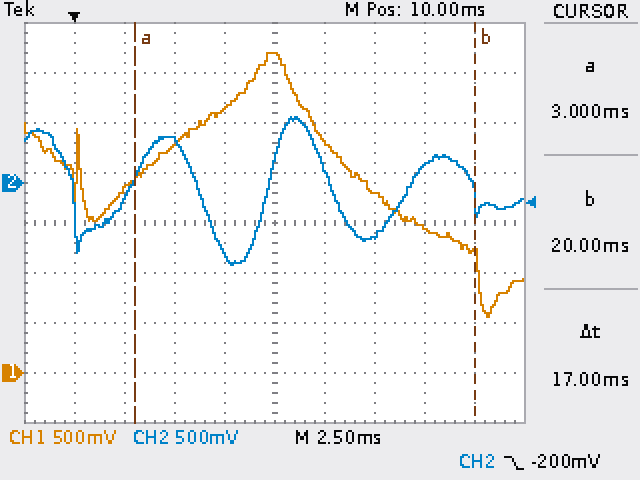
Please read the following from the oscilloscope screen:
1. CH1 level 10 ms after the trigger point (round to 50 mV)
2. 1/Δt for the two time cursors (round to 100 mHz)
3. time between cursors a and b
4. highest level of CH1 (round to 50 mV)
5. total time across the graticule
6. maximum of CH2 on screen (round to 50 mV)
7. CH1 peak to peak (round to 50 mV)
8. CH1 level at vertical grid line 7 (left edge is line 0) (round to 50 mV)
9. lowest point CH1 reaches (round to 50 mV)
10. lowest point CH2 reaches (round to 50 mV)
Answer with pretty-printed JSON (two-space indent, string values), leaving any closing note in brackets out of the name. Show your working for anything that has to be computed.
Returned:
{
  "CH1 level 10 ms after the trigger point": "3.20 V",
  "1/Δt for the two time cursors": "1 / 17 ms ≈ 58.8 Hz",
  "time between cursors a and b": "17 ms",
  "highest level of CH1": "3.20 V",
  "total time across the graticule": "25 ms",
  "maximum of CH2 on screen": "650 mV",
  "CH1 peak to peak": "3.20 V − (550 mV) = 2.65 V",
  "CH1 level at vertical grid line 7 (left edge is line 0)": "1.80 V",
  "lowest point CH1 reaches": "550 mV",
  "lowest point CH2 reaches": "-800 mV"
}
